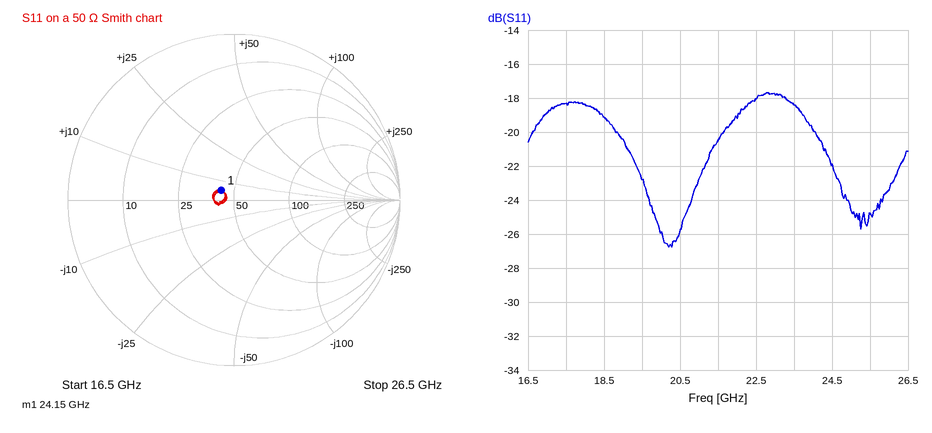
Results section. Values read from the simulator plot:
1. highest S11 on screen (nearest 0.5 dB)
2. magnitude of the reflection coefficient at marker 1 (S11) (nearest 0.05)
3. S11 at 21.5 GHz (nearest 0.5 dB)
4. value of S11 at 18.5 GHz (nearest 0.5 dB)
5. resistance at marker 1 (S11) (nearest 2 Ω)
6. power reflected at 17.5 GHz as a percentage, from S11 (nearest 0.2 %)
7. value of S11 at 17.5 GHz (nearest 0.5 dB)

-17.5 dB
0.10
-20.5 dB
-19.0 dB
42 Ω
1.4 %
-18.5 dB
